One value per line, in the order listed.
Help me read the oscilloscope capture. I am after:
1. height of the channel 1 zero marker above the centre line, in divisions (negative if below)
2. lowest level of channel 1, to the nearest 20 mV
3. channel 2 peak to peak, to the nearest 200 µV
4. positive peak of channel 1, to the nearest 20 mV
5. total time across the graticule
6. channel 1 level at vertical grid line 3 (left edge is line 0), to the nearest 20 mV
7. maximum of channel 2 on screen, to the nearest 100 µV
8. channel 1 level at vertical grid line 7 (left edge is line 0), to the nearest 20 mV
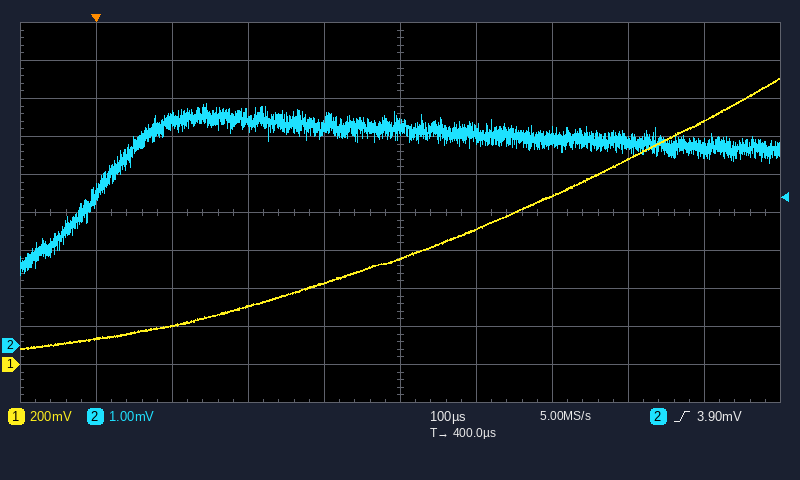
-4.0 div
80 mV
4.6 mV
1.50 V
1 ms
300 mV
6.4 mV
880 mV
